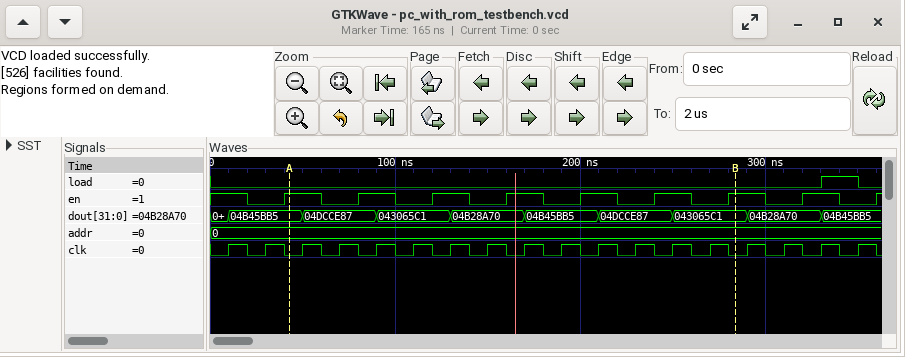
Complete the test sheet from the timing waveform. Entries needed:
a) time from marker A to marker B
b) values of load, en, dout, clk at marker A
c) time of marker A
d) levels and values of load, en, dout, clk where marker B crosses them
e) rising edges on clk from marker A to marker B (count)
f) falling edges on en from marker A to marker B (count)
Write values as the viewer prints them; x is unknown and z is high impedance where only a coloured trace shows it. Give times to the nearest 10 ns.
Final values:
240 ns
load=0, en=1, dout=04B45BB5, clk=0
40 ns
load=0, en=1, dout=043065C1, clk=0
12
6
